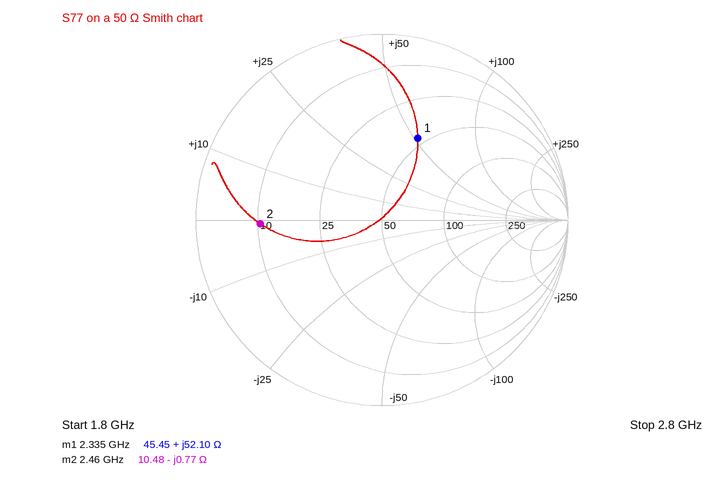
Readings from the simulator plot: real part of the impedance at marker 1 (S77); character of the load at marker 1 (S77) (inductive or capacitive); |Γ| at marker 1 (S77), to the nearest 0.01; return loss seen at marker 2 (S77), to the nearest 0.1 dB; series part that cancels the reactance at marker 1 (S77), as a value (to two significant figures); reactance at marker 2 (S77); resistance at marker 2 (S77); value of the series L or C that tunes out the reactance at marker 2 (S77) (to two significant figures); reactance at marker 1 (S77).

45.45 Ω
inductive
0.48
3.7 dB
1.3 pF
-0.77 Ω
10.48 Ω
50 pH
+52.10 Ω
